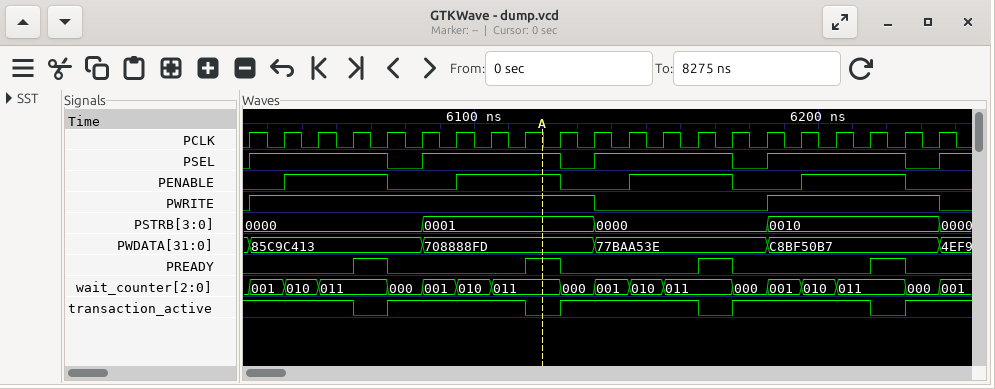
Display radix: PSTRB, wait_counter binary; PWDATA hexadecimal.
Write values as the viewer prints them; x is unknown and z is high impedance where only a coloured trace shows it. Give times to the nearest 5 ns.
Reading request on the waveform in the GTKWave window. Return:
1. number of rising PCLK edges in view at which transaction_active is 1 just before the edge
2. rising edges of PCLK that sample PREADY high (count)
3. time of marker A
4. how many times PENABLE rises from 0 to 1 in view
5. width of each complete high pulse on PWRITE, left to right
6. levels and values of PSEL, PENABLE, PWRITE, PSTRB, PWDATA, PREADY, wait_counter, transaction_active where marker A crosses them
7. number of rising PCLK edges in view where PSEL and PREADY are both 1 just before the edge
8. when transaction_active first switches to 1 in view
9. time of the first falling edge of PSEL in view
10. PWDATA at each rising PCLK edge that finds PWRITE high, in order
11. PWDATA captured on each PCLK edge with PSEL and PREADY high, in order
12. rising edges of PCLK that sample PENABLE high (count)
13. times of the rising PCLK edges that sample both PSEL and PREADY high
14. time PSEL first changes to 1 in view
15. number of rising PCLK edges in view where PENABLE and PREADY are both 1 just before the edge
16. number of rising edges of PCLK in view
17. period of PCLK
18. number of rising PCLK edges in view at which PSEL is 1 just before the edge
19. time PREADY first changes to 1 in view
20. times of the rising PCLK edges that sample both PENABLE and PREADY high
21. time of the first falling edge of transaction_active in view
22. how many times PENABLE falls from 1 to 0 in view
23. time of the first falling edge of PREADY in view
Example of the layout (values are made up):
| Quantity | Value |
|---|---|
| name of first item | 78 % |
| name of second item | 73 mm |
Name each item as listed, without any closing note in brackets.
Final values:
| Quantity | Value |
|---|---|
| number of rising PCLK edges in view at which transaction_active is 1 just before the edge | 17 |
| rising edges of PCLK that sample PREADY high | 4 |
| time of marker A | 6120 ns |
| how many times PENABLE rises from 0 to 1 in view | 4 |
| width of each complete high pulse on PWRITE, left to right | 100 ns, 50 ns |
| levels and values of PSEL, PENABLE, PWRITE, PSTRB, PWDATA, PREADY, wait_counter, transaction_active where marker A crosses them | PSEL=1, PENABLE=1, PWRITE=1, PSTRB=0001, PWDATA=708888FD, PREADY=1, wait_counter=011, transaction_active=0 |
| number of rising PCLK edges in view where PSEL and PREADY are both 1 just before the edge | 4 |
| when transaction_active first switches to 1 in view | 6075 ns |
| time of the first falling edge of PSEL in view | 6075 ns |
| PWDATA at each rising PCLK edge that finds PWRITE high, in order | 85C9C413, 85C9C413, 85C9C413, 85C9C413, 85C9C413, 708888FD, 708888FD, 708888FD, 708888FD, 708888FD, C8BF50B7, C8BF50B7, C8BF50B7, C8BF50B7, C8BF50B7 |
| PWDATA captured on each PCLK edge with PSEL and PREADY high, in order | 85C9C413, 708888FD, 77BAA53E, C8BF50B7 |
| rising edges of PCLK that sample PENABLE high | 12 |
| times of the rising PCLK edges that sample both PSEL and PREADY high | 6075 ns, 6125 ns, 6175 ns, 6225 ns |
| time PSEL first changes to 1 in view | 6035 ns |
| number of rising PCLK edges in view where PENABLE and PREADY are both 1 just before the edge | 4 |
| number of rising edges of PCLK in view | 21 |
| period of PCLK | 10 ns |
| number of rising PCLK edges in view at which PSEL is 1 just before the edge | 16 |
| time PREADY first changes to 1 in view | 6065 ns |
| times of the rising PCLK edges that sample both PENABLE and PREADY high | 6075 ns, 6125 ns, 6175 ns, 6225 ns |
| time of the first falling edge of transaction_active in view | 6065 ns |
| how many times PENABLE falls from 1 to 0 in view | 4 |
| time of the first falling edge of PREADY in view | 6075 ns |
